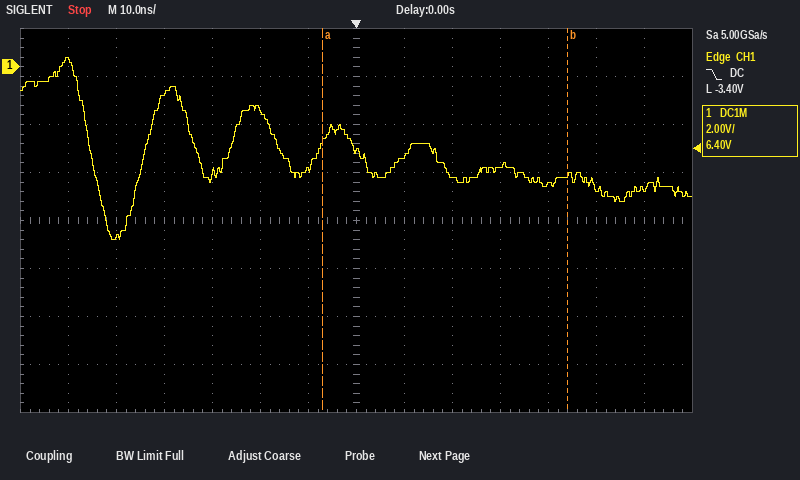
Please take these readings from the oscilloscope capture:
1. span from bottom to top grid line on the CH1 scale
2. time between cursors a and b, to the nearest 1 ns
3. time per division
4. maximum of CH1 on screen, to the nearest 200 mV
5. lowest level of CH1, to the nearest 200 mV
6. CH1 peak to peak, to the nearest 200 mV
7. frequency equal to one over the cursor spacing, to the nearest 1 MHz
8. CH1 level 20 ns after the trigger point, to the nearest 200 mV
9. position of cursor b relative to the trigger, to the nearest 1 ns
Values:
16 V
51 ns
10 ns
400 mV
-7.2 V
7.6 V
20 MHz
-4.6 V
+44 ns
